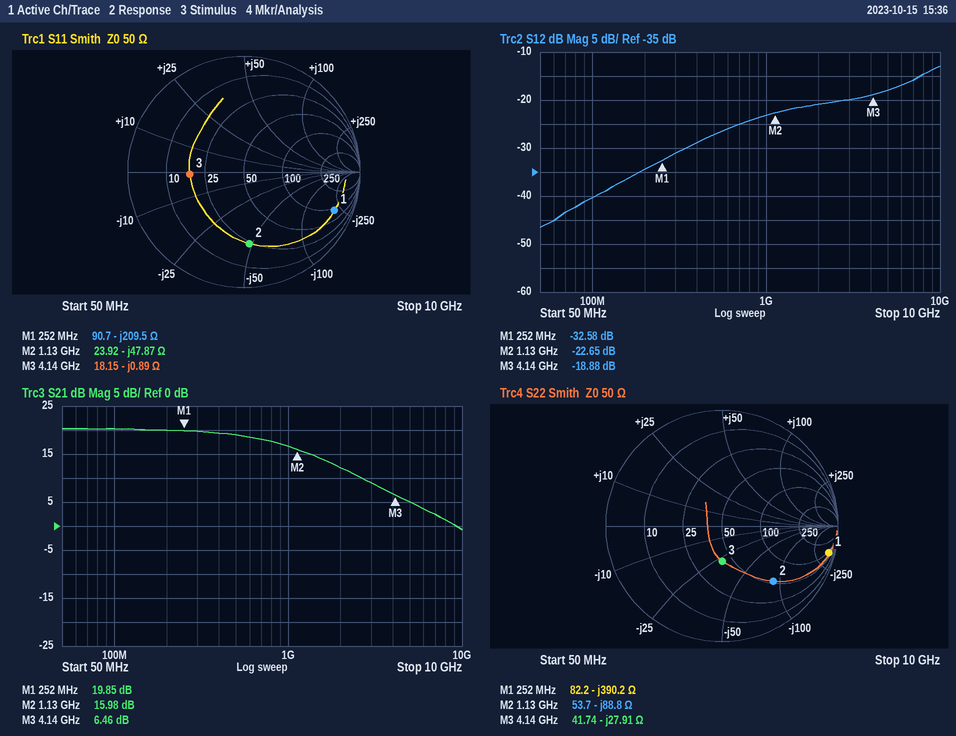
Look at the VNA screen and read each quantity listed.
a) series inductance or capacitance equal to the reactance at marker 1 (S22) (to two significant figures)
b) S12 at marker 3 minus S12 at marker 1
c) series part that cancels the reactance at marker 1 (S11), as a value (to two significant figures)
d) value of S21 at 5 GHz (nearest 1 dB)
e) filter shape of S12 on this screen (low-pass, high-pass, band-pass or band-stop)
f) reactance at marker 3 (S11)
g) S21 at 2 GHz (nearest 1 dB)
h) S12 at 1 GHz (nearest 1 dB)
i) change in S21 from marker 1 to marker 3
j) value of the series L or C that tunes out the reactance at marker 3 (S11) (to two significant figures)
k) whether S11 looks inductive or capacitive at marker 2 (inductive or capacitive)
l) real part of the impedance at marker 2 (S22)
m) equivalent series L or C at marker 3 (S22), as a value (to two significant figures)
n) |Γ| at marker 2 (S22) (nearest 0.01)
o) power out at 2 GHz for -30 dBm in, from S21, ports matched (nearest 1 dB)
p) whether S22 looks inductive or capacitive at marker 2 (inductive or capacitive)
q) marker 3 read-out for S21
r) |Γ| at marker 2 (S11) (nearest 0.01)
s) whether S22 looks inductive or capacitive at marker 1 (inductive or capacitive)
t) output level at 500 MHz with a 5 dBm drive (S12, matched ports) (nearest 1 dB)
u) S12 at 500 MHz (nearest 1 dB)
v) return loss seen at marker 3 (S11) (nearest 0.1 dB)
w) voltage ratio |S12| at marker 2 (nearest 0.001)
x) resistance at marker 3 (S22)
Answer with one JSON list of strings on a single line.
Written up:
["1.6 pF", "13.70 dB", "130 nH", "5 dB", "high-pass", "-0.89 Ω", "12 dB", "-23 dB", "-13.39 dB", "34 pH", "capacitive", "53.7 Ω", "1.4 pF", "0.65", "-18 dBm", "capacitive", "6.46 dB", "0.62", "capacitive", "-22 dBm", "-27 dB", "6.6 dB", "0.074", "41.74 Ω"]
